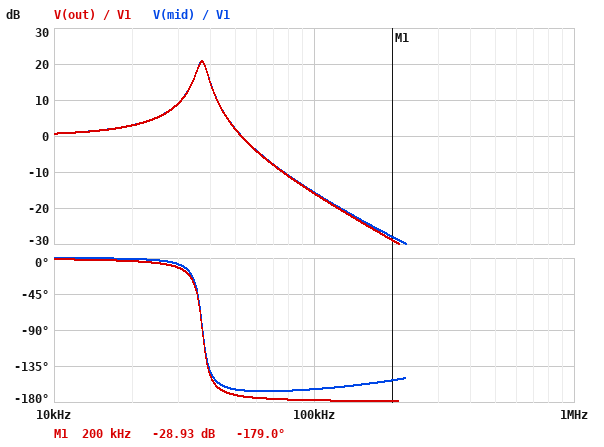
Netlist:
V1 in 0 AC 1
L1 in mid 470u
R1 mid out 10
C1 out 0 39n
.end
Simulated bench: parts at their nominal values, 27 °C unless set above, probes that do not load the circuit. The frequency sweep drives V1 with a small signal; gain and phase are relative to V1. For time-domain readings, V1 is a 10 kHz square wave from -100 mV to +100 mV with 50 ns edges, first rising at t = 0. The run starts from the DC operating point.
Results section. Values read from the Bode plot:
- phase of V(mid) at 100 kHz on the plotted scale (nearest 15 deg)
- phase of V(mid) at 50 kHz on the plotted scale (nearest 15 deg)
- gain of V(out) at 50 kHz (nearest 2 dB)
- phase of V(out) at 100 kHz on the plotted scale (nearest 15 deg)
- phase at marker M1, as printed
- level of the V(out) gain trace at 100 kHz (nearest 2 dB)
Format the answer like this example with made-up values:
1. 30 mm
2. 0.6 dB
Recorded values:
1. -165 deg
2. -165 deg
3. 2 dB
4. -180 deg
5. -179.0 deg
6. -16 dB
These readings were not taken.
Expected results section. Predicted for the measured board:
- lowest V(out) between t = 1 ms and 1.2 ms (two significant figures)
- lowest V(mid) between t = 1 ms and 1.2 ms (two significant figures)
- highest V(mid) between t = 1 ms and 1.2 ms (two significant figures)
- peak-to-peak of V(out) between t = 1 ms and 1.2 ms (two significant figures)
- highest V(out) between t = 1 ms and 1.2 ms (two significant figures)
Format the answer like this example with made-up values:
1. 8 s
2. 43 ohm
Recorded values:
1. -220 mV
2. -220 mV
3. 220 mV
4. 440 mV
5. 220 mV
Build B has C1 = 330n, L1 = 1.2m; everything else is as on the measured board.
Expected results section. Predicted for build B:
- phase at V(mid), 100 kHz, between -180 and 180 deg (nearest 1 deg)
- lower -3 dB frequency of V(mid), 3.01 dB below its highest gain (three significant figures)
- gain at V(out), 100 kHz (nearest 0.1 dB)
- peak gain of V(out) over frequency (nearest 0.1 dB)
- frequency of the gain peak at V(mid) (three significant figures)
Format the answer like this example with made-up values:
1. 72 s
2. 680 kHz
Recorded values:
1. -115 deg
2. 7.25 kHz
3. -43.8 dB
4. 15.6 dB
5. 7.94 kHz
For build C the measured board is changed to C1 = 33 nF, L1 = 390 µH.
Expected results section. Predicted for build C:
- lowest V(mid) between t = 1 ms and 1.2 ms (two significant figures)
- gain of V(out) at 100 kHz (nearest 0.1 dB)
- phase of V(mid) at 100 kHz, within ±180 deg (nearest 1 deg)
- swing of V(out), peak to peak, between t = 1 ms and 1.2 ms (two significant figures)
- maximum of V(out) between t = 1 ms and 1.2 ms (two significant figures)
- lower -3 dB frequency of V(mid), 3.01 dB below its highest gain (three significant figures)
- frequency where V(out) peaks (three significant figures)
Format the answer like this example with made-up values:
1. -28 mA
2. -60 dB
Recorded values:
1. -240 mV
2. -12.2 dB
3. -165 deg
4. 480 mV
5. 240 mV
6. 42.2 kHz
7. 44.3 kHz
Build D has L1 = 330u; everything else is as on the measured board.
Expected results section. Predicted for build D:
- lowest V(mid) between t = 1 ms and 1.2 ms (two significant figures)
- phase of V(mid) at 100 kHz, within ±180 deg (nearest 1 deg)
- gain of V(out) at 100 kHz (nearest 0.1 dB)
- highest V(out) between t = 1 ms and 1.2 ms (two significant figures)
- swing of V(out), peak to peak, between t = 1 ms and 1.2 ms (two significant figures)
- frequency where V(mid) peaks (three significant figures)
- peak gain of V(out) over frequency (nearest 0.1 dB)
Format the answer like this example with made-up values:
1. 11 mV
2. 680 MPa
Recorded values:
1. -240 mV
2. -163 deg
3. -12.2 dB
4. 240 mV
5. 480 mV
6. 44.2 kHz
7. 19.3 dB
